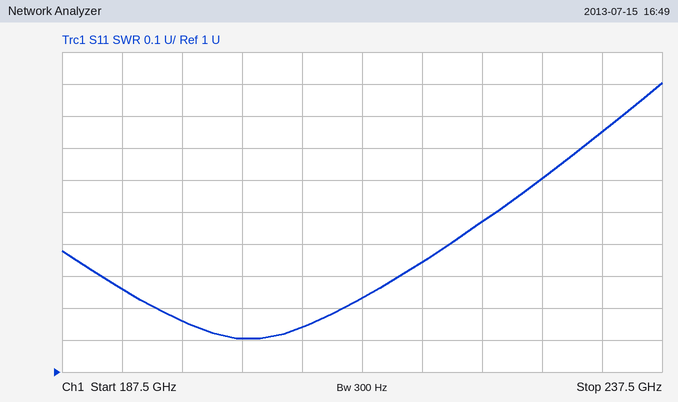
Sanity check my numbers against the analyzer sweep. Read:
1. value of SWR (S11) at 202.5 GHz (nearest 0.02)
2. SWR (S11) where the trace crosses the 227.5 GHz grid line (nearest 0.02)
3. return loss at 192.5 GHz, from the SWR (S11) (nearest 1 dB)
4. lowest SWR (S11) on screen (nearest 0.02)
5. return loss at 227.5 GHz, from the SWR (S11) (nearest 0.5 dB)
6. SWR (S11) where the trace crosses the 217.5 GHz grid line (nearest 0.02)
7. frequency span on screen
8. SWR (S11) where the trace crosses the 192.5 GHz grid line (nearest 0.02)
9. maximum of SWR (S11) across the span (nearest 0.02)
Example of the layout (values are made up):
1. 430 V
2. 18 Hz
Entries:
1. 1.10
2. 1.60
3. 19 dB
4. 1.10
5. 12.5 dB
6. 1.34
7. 50 GHz
8. 1.26
9. 1.90
